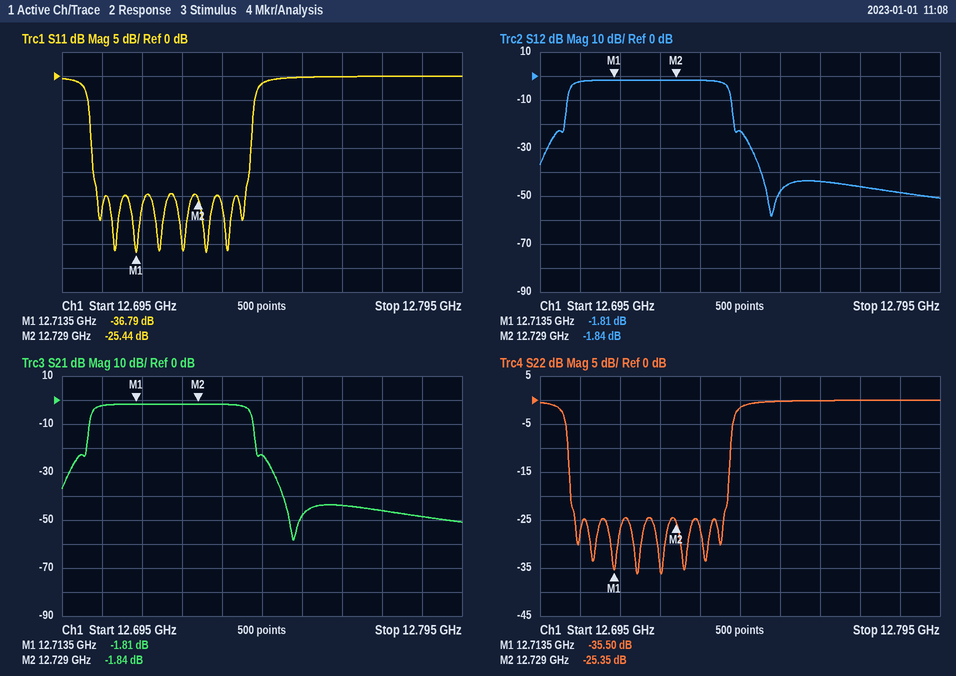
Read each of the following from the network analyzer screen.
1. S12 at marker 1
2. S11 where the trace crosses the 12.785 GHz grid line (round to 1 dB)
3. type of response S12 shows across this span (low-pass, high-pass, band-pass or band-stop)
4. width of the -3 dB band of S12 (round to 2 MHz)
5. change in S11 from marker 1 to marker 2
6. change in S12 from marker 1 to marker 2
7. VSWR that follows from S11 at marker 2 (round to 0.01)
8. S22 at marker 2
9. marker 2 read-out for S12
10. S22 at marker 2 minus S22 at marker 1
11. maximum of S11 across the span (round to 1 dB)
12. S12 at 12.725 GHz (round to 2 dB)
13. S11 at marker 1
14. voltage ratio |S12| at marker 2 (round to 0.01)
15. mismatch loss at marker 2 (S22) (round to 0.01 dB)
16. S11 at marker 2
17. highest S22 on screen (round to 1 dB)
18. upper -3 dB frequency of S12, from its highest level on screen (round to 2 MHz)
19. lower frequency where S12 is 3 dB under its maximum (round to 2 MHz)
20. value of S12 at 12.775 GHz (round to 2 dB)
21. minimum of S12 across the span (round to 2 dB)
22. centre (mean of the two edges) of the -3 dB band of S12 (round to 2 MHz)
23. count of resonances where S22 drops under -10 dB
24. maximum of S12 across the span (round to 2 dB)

-1.81 dB
0 dB
band-pass
40 MHz
11.35 dB
-0.03 dB
1.11
-25.35 dB
-1.84 dB
10.15 dB
0 dB
-2 dB
-36.79 dB
0.81
0.01 dB
-25.44 dB
0 dB
12.742 GHz
12.702 GHz
-46 dB
-58 dB
12.722 GHz
8
-2 dB
